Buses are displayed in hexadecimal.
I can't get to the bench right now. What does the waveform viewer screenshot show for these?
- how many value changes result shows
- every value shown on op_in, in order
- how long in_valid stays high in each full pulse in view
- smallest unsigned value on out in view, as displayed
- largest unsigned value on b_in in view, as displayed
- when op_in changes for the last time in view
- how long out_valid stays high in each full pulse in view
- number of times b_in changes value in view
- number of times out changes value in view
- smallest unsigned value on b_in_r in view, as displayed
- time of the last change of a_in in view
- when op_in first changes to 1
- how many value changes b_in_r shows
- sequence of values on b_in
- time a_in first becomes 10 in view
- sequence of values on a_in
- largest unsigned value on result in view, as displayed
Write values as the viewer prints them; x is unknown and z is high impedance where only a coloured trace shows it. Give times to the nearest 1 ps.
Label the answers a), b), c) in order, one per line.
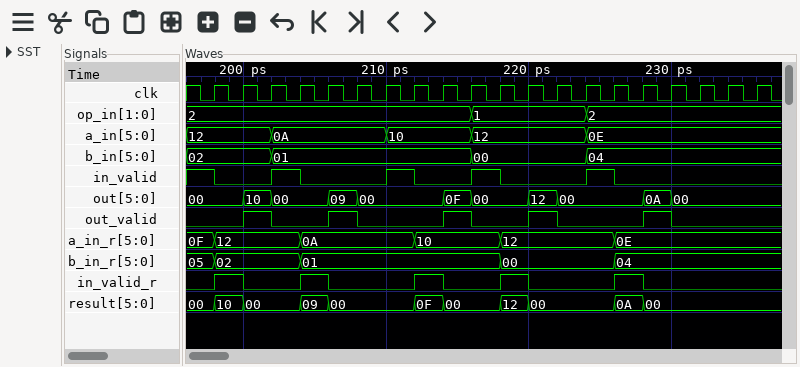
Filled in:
a) 10
b) 2, 1, 2
c) 2 ps, 2 ps, 2 ps, 2 ps
d) 00
e) 04
f) 224 ps
g) 2 ps, 2 ps, 2 ps, 2 ps, 2 ps
h) 3
i) 10
j) 00
k) 224 ps
l) 216 ps
m) 4
n) 02, 01, 00, 04
o) 210 ps
p) 12, 0A, 10, 12, 0E
q) 12
